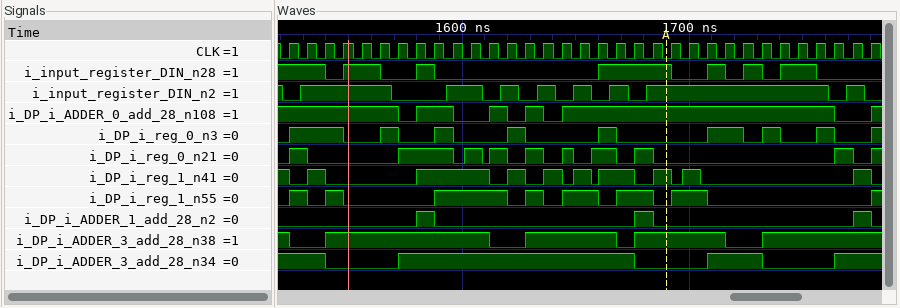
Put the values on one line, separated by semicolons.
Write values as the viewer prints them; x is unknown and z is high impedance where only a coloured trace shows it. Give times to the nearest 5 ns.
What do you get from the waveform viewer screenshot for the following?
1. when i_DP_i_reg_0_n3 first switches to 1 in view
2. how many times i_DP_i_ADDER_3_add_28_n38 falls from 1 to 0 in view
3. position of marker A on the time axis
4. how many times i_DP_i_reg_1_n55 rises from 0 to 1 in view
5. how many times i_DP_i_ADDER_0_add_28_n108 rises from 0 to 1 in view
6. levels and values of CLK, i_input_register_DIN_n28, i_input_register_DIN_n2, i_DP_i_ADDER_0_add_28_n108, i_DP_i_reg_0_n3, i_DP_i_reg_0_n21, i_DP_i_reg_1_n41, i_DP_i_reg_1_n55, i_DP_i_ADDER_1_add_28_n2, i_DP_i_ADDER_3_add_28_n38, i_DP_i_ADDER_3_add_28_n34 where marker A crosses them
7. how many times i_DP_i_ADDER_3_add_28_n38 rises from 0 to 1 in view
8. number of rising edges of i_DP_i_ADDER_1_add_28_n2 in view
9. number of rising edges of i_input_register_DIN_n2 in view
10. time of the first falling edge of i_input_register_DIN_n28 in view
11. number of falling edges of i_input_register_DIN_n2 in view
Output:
1525 ns; 4; 1690 ns; 8; 5; CLK=0, i_input_register_DIN_n28=1, i_input_register_DIN_n2=1, i_DP_i_ADDER_0_add_28_n108=1, i_DP_i_reg_0_n3=0, i_DP_i_reg_0_n21=0, i_DP_i_reg_1_n41=1, i_DP_i_reg_1_n55=0, i_DP_i_ADDER_1_add_28_n2=0, i_DP_i_ADDER_3_add_28_n38=1, i_DP_i_ADDER_3_add_28_n34=0; 4; 3; 8; 1540 ns; 9
